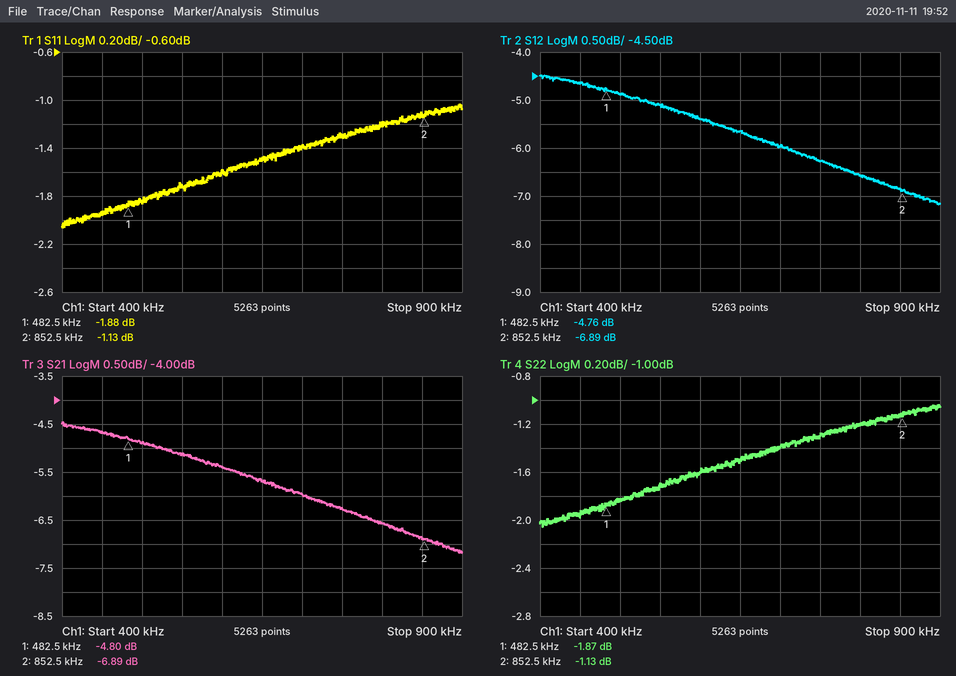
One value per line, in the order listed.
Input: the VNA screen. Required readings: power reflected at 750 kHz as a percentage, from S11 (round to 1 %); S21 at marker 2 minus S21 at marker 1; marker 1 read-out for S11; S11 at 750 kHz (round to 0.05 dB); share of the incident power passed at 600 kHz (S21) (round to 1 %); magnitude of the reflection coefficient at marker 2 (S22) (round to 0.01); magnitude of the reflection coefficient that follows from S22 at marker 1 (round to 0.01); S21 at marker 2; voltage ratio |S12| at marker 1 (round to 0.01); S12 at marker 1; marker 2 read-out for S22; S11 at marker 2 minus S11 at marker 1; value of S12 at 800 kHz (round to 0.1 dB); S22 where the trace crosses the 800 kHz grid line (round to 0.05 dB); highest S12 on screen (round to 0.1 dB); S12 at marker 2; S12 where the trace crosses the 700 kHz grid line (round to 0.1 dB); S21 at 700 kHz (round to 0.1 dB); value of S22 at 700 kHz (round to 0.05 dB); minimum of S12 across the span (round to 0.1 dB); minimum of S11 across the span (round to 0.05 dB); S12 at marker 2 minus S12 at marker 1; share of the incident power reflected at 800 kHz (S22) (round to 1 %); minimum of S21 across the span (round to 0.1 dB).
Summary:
74 %
-2.09 dB
-1.88 dB
-1.30 dB
29 %
0.88
0.81
-6.89 dB
0.58
-4.76 dB
-1.13 dB
0.75 dB
-6.6 dB
-1.20 dB
-4.5 dB
-6.89 dB
-6.0 dB
-6.0 dB
-1.40 dB
-7.2 dB
-2.05 dB
-2.13 dB
76 %
-7.2 dB
